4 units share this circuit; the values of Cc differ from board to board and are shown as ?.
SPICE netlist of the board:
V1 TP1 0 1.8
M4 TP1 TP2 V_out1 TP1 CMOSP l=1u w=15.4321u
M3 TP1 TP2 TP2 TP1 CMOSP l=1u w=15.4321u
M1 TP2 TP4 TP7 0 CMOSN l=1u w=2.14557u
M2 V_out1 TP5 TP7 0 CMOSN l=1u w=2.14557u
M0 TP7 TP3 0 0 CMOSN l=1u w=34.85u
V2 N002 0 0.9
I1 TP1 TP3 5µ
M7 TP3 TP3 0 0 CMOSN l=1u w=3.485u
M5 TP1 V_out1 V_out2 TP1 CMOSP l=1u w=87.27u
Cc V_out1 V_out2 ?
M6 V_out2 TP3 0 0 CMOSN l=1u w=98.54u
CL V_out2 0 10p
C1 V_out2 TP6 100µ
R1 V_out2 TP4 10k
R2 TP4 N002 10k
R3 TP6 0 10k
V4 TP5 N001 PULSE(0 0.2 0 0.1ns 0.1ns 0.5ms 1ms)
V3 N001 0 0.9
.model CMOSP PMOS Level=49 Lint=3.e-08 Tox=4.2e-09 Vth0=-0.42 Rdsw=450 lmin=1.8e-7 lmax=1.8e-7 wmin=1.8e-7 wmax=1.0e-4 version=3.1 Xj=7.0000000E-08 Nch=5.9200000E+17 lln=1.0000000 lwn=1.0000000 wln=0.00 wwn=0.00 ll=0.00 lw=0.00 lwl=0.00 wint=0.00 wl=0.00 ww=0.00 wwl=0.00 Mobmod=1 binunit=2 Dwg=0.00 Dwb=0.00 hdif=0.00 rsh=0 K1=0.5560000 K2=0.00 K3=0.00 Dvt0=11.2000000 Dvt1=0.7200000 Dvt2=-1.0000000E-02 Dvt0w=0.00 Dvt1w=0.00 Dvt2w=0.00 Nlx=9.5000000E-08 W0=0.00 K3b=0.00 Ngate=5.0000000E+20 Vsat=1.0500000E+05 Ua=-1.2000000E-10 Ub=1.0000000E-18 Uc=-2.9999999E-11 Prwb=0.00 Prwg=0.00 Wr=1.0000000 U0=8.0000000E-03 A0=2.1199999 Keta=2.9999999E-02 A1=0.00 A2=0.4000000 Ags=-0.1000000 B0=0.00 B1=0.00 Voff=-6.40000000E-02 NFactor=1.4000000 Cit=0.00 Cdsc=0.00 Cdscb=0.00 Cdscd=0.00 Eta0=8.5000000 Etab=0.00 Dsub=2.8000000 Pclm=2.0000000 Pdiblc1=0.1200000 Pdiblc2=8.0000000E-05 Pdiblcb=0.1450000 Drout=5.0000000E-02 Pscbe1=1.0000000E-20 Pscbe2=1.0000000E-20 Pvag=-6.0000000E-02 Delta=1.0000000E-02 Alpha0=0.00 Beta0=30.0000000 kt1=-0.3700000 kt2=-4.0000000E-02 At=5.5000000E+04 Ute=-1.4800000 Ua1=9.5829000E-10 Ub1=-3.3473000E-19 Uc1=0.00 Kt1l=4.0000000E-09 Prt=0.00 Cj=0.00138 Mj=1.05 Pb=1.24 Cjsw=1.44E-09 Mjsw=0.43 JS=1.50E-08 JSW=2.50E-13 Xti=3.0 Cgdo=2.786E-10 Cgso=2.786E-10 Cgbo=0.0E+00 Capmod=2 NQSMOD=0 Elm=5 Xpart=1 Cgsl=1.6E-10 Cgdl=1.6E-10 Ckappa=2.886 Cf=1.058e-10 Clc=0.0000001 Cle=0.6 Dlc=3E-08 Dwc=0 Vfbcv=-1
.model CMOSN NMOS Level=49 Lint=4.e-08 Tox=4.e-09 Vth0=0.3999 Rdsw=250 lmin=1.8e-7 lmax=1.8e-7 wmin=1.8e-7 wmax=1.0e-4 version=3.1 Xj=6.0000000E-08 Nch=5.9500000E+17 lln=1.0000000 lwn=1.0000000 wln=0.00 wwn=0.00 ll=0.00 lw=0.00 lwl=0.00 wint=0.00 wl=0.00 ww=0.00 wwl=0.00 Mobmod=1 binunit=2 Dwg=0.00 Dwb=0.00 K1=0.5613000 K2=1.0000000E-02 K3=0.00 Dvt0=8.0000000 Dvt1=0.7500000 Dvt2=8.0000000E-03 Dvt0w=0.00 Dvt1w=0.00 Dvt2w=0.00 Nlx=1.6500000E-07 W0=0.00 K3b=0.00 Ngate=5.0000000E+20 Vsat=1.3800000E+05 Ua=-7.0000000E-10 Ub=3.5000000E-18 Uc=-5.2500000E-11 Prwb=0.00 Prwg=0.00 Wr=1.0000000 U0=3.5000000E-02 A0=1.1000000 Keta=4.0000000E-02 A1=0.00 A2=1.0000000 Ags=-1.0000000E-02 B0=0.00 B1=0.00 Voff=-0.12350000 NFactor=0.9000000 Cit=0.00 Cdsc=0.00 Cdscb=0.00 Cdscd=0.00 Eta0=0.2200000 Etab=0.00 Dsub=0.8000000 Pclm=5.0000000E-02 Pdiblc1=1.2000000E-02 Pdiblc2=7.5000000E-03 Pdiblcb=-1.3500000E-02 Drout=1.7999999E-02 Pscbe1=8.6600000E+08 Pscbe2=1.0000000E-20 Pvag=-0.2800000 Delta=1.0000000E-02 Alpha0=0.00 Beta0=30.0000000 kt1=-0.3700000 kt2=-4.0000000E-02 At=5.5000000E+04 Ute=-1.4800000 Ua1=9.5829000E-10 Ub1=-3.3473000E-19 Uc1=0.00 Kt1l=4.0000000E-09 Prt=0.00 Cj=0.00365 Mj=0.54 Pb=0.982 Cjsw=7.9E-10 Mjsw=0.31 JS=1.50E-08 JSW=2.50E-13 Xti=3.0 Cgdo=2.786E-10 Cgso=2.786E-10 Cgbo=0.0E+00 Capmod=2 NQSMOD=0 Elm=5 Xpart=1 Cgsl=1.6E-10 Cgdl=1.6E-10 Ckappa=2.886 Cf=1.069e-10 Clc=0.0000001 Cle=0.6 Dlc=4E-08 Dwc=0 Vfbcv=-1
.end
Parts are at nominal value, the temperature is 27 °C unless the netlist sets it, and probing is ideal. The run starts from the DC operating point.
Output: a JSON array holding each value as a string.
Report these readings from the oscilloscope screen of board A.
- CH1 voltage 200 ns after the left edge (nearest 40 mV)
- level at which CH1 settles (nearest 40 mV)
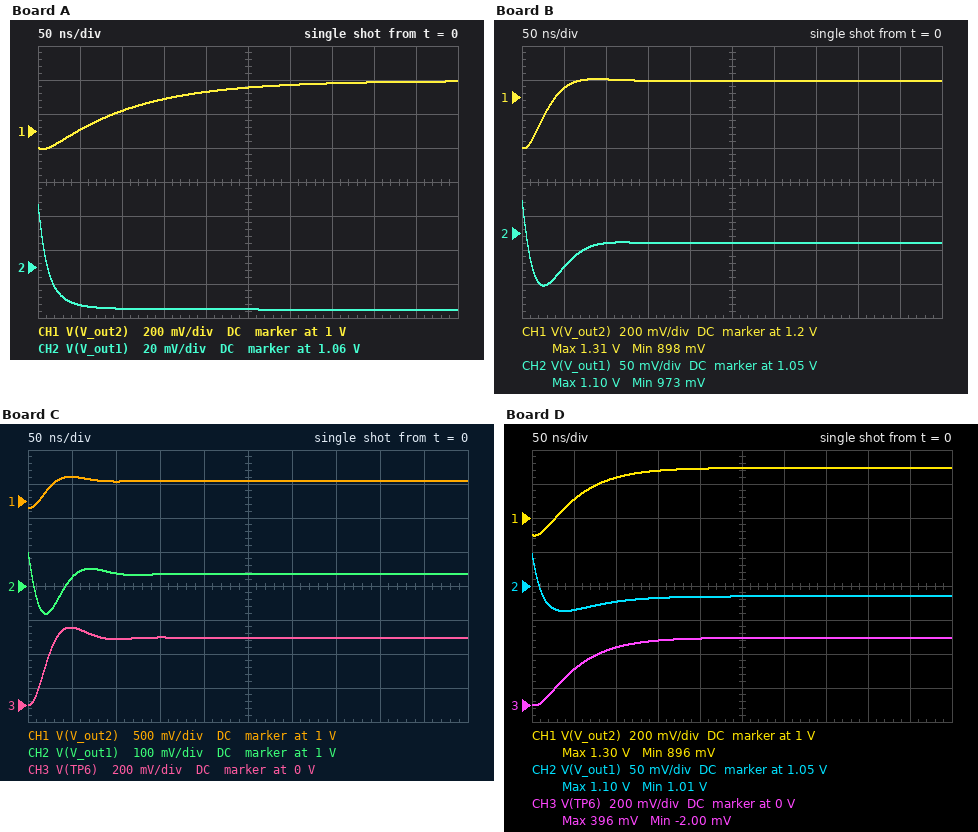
["1.24 V", "1.28 V"]
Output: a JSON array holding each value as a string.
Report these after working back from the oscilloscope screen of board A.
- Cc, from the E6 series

["6.8 pF"]
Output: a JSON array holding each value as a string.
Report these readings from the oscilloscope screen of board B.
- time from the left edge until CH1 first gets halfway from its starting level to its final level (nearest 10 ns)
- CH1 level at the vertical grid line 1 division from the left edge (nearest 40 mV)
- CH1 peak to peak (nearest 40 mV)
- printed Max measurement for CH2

["30 ns", "1.24 V", "400 mV", "1.10 V"]
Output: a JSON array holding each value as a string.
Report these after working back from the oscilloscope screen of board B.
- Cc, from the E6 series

["1.5 pF"]
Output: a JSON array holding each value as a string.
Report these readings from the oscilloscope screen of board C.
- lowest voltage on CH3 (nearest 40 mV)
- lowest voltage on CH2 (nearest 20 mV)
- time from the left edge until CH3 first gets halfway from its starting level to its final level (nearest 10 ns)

["0 V", "920 mV", "20 ns"]
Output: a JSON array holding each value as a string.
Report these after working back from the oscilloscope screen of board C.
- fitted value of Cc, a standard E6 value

["680 fF"]
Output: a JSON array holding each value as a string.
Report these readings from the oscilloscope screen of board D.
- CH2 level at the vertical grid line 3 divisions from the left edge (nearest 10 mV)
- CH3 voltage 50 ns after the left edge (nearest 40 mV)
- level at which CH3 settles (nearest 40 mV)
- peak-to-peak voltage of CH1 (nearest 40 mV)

["1.03 V", "200 mV", "400 mV", "400 mV"]
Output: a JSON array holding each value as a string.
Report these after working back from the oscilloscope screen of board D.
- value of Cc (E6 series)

["3.3 pF"]
